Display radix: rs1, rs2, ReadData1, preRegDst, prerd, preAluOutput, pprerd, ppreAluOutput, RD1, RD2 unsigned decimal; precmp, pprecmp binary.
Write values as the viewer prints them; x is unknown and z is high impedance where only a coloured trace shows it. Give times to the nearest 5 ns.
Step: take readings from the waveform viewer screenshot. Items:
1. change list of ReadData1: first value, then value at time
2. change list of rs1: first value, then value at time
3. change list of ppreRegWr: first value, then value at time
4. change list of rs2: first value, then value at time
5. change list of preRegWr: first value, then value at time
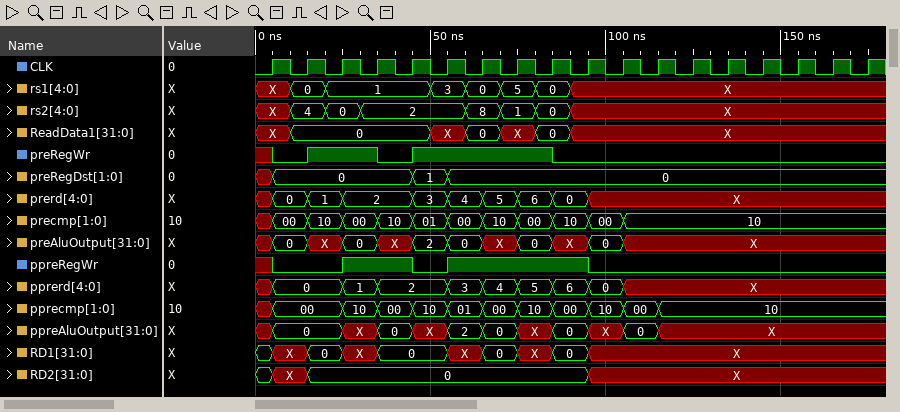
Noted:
X, 0 at 10 ns, X at 50 ns, 0 at 60 ns, X at 70 ns, 0 at 80 ns, X at 90 ns
X, 0 at 10 ns, 1 at 20 ns, 3 at 50 ns, 0 at 60 ns, 5 at 70 ns, 0 at 80 ns, X at 90 ns
x, 0 at 5 ns, 1 at 25 ns, 0 at 45 ns, 1 at 55 ns, 0 at 95 ns
X, 4 at 10 ns, 0 at 20 ns, 2 at 30 ns, 8 at 60 ns, 1 at 70 ns, 0 at 80 ns, X at 90 ns
x, 0 at 5 ns, 1 at 15 ns, 0 at 35 ns, 1 at 45 ns, 0 at 85 ns
